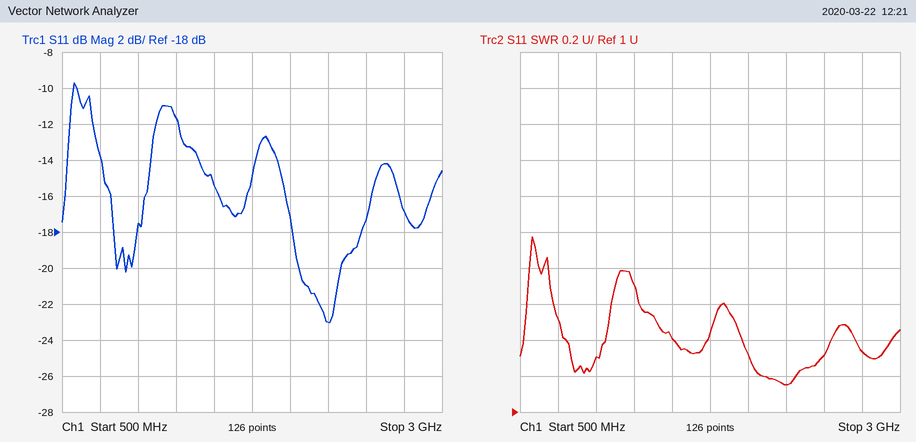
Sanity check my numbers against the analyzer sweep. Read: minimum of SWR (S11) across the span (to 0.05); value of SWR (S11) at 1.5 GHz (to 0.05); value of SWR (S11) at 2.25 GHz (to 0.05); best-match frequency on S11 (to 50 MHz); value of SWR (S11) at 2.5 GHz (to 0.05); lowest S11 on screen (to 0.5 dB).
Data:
1.15
1.40
1.15
2.25 GHz
1.30
-23.0 dB
